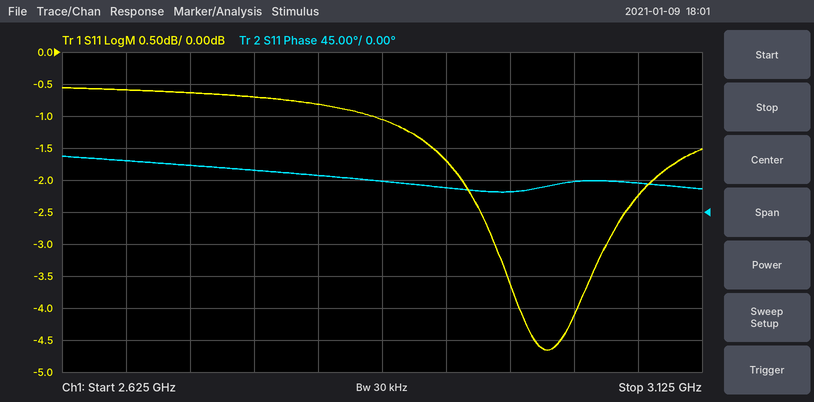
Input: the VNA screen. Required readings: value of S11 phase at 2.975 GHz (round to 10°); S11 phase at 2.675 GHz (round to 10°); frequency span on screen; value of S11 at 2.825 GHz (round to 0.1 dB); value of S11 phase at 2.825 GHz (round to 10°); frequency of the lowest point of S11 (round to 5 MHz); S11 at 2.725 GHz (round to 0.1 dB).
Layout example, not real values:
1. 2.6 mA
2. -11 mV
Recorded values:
1. 30°
2. 70°
3. 500 MHz
4. -0.8 dB
5. 50°
6. 3.005 GHz
7. -0.6 dB
